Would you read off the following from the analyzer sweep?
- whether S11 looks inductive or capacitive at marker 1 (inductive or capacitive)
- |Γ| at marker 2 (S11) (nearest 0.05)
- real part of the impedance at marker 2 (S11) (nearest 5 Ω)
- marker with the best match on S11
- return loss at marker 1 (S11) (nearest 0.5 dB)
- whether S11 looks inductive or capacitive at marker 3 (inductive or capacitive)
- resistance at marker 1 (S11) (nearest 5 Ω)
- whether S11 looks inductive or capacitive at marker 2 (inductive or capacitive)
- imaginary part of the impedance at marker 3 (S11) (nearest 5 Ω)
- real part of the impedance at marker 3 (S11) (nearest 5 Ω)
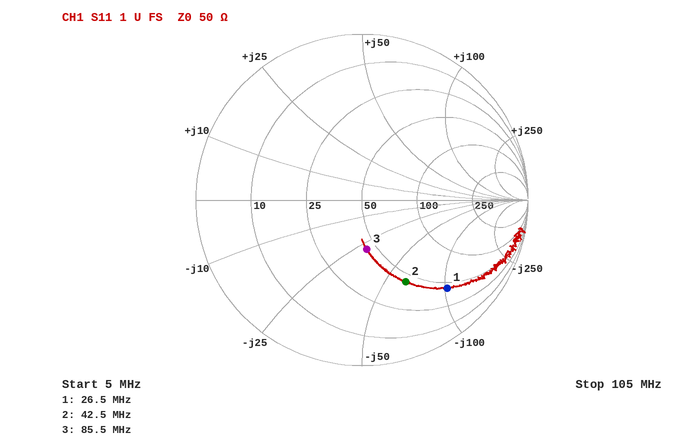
capacitive
0.55
45 Ω
marker 3
2.5 dB
capacitive
45 Ω
capacitive
-30 Ω
45 Ω
